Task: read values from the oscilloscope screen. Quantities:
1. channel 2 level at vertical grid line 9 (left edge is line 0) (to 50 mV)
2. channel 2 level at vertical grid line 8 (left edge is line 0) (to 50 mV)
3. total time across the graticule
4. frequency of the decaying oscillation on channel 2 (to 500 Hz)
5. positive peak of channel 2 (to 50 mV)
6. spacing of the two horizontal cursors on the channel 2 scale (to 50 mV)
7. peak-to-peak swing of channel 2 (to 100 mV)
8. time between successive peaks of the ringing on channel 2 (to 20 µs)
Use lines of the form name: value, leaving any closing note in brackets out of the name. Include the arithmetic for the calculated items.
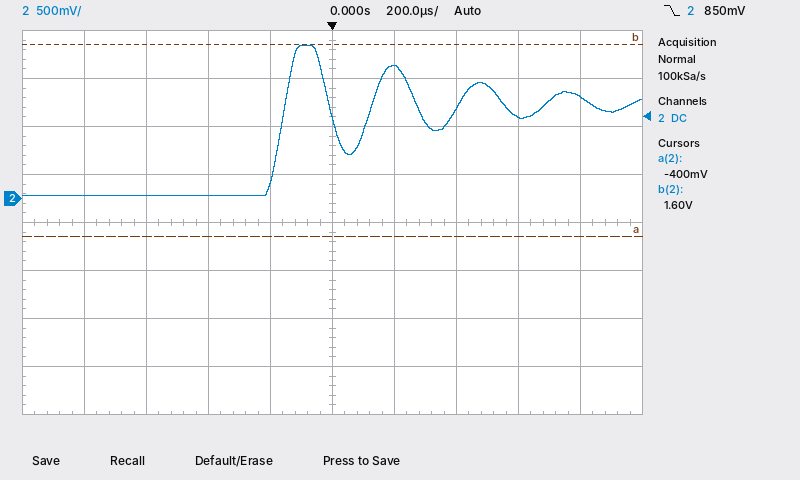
channel 2 level at vertical grid line 9 (left edge is line 0): 1.05 V
channel 2 level at vertical grid line 8 (left edge is line 0): 850 mV
total time across the graticule: 2 ms
frequency of the decaying oscillation on channel 2: 1 / 280 µs ≈ 3.57 kHz, so 3.5 kHz to the nearest 500 Hz
positive peak of channel 2: 1.60 V
spacing of the two horizontal cursors on the channel 2 scale: 2.00 V
peak-to-peak swing of channel 2: 1.60 V
time between successive peaks of the ringing on channel 2: 280 µs
